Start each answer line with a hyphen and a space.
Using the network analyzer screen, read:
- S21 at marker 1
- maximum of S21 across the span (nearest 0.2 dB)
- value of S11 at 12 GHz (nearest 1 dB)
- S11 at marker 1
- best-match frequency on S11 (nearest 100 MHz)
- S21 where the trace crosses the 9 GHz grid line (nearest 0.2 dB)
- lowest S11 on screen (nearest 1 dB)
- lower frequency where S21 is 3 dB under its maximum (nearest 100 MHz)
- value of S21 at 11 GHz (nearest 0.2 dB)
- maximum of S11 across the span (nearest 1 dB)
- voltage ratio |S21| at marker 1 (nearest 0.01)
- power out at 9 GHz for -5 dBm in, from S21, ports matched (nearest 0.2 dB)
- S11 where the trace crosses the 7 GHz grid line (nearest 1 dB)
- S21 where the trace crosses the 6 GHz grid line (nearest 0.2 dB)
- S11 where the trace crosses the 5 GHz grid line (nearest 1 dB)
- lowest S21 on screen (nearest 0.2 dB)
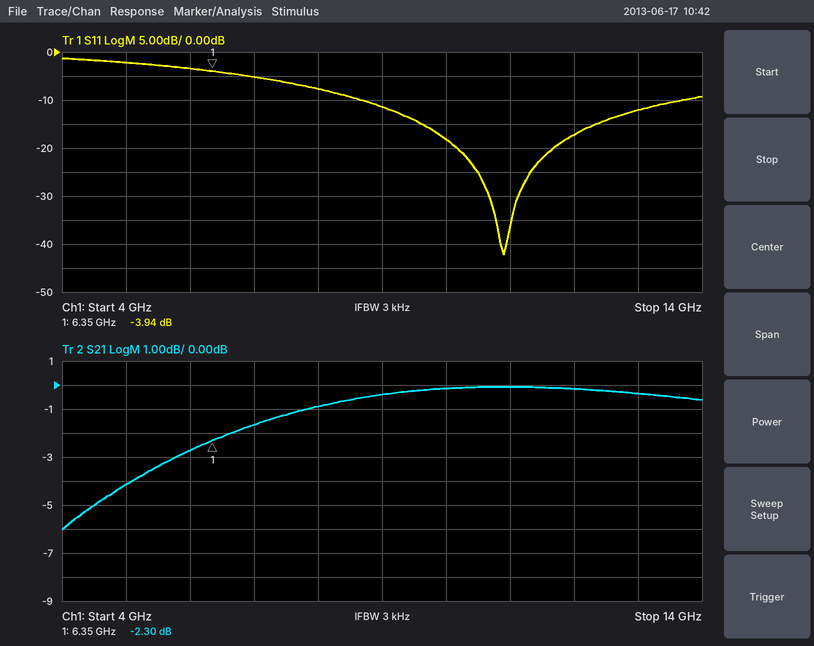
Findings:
- -2.30 dB
- 0.0 dB
- -17 dB
- -3.94 dB
- 10.9 GHz
- -0.4 dB
- -42 dB
- 5.7 GHz
- 0.0 dB
- -1 dB
- 0.77
- -5.4 dBm
- -5 dB
- -2.8 dB
- -2 dB
- -6.0 dB
